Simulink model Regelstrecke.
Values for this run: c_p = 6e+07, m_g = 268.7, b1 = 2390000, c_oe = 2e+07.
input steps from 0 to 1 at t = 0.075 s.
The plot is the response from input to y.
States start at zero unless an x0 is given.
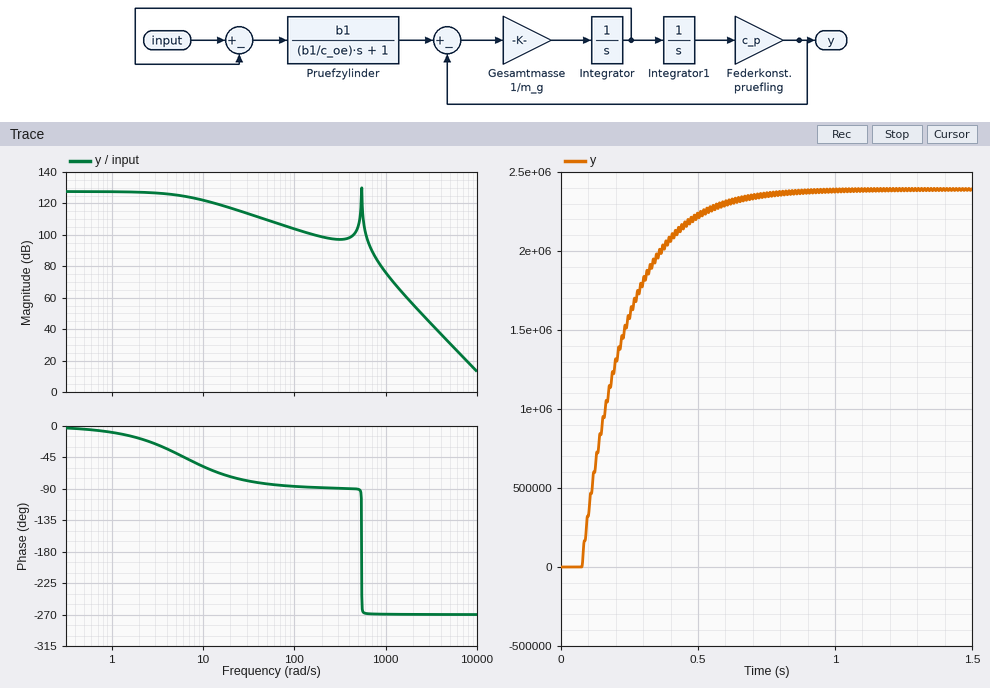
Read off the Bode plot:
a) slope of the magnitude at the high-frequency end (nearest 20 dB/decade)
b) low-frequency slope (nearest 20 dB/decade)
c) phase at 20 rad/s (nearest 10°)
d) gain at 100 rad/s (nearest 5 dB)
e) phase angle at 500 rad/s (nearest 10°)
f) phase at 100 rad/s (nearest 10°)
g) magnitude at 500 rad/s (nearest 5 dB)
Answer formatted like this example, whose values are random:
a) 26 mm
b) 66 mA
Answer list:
a) -60 dB/decade
b) 0 dB/decade
c) -70°
d) 105 dB
e) -90°
f) -90°
g) 105 dB
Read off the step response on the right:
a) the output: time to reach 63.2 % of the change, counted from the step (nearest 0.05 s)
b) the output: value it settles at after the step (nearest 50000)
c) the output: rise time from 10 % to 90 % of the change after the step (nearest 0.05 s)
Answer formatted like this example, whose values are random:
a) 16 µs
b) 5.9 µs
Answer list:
a) 0.15 s
b) 2400000
c) 0.35 s
